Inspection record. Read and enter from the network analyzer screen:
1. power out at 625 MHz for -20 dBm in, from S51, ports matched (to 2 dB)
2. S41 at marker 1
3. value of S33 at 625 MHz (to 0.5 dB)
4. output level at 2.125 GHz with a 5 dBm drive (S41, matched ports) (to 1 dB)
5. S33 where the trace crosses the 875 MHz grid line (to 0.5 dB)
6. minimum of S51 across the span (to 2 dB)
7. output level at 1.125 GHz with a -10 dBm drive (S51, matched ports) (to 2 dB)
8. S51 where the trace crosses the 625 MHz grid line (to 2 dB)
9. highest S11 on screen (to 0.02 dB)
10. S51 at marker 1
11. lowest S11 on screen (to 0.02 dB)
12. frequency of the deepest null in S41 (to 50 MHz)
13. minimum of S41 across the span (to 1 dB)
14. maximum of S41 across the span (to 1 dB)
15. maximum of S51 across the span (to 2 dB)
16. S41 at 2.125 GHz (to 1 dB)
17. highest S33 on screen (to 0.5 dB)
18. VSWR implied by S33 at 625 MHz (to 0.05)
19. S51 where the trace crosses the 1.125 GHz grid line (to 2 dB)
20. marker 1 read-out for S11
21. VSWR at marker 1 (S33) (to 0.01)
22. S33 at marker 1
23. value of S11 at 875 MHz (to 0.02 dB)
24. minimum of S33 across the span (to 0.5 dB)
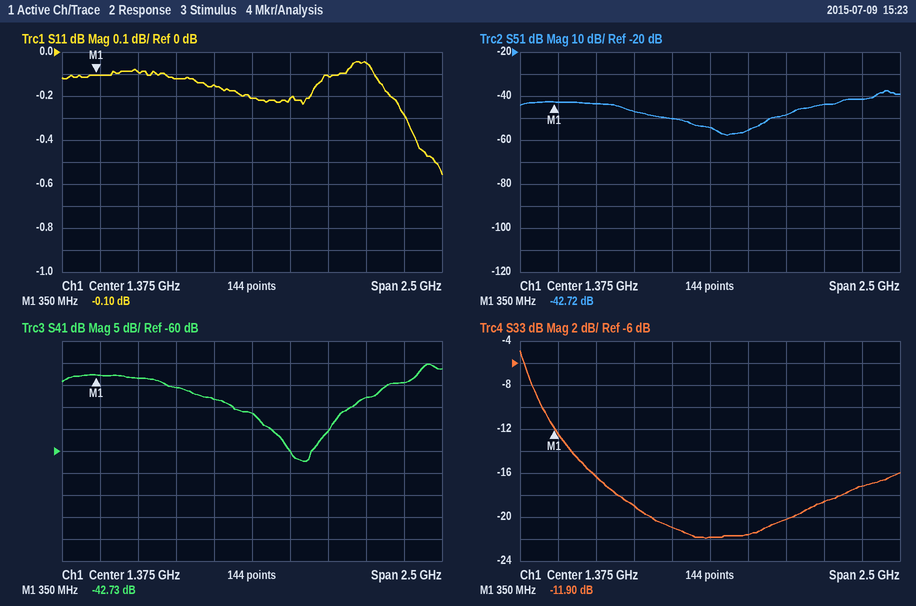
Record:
-64 dBm
-42.73 dB
-16.5 dB
-43 dBm
-19.0 dB
-58 dB
-60 dBm
-44 dB
-0.04 dB
-42.72 dB
-0.56 dB
1.70 GHz
-62 dB
-40 dB
-38 dB
-48 dB
-5.0 dB
1.35
-50 dB
-0.10 dB
1.68
-11.90 dB
-0.12 dB
-22.0 dB
